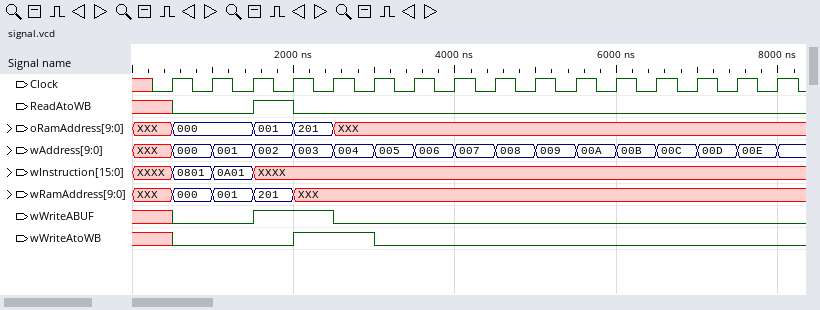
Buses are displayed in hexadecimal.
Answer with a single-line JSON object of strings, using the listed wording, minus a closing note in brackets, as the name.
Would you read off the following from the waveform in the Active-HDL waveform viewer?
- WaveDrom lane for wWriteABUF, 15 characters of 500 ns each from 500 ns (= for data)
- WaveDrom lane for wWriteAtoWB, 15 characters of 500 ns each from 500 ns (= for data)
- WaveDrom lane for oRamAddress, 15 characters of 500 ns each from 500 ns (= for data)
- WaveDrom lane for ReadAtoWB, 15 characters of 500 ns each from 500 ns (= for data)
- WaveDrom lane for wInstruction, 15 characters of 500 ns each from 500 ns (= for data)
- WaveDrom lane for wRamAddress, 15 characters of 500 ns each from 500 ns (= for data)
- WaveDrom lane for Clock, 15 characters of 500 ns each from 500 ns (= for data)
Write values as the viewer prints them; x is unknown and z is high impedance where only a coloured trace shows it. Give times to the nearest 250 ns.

{"WaveDrom lane for wWriteABUF, 15 characters of 500 ns each from 500 ns": "{name: 'wWriteABUF', wave: '0.1.0..........'}", "WaveDrom lane for wWriteAtoWB, 15 characters of 500 ns each from 500 ns": "{name: 'wWriteAtoWB', wave: '0..1.0.........'}", "WaveDrom lane for oRamAddress, 15 characters of 500 ns each from 500 ns": "{name: 'oRamAddress', wave: '=.==x..........', data: '000 001 201'}", "WaveDrom lane for ReadAtoWB, 15 characters of 500 ns each from 500 ns": "{name: 'ReadAtoWB', wave: '0.10...........'}", "WaveDrom lane for wInstruction, 15 characters of 500 ns each from 500 ns": "{name: 'wInstruction', wave: '==x............', data: '0801 0A01'}", "WaveDrom lane for wRamAddress, 15 characters of 500 ns each from 500 ns": "{name: 'wRamAddress', wave: '===x...........', data: '000 001 201'}", "WaveDrom lane for Clock, 15 characters of 500 ns each from 500 ns": "{name: 'Clock', wave: 'p..............'}"}
